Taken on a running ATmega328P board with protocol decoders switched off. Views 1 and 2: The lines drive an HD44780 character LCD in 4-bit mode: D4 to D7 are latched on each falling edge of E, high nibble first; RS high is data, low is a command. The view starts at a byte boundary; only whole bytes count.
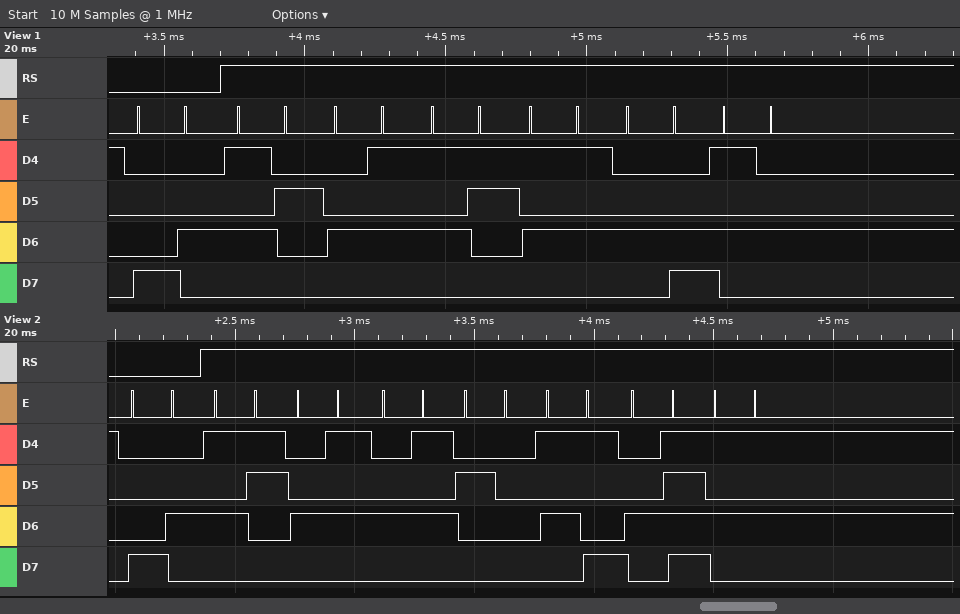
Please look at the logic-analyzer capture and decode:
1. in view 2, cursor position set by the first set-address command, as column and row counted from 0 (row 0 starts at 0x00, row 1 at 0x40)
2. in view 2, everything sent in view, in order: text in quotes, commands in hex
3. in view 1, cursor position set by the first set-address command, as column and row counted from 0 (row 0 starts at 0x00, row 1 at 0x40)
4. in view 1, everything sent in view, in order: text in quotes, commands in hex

column 4, row 0
0x84 "SEE YOU"
column 4, row 0
0x84 "RESULT"
